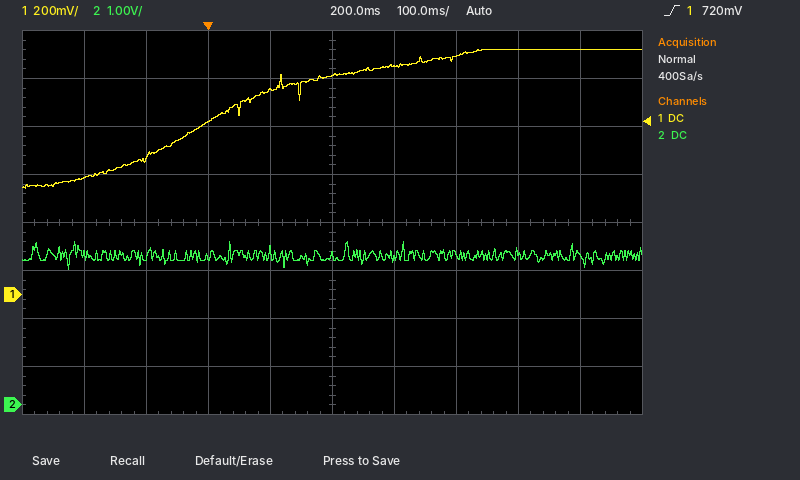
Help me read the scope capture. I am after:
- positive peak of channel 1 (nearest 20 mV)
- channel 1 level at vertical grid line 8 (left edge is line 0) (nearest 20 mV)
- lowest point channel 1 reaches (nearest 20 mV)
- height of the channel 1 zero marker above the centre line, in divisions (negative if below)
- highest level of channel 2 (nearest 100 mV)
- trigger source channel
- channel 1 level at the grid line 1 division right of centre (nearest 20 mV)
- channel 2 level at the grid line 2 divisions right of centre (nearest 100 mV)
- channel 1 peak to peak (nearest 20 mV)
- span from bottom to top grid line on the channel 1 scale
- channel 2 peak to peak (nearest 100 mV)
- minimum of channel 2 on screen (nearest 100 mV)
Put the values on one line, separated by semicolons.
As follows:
1.02 V; 1.02 V; 440 mV; -1.5 div; 3.4 V; channel 1; 960 mV; 3.1 V; 580 mV; 1.6 V; 600 mV; 2.8 V
